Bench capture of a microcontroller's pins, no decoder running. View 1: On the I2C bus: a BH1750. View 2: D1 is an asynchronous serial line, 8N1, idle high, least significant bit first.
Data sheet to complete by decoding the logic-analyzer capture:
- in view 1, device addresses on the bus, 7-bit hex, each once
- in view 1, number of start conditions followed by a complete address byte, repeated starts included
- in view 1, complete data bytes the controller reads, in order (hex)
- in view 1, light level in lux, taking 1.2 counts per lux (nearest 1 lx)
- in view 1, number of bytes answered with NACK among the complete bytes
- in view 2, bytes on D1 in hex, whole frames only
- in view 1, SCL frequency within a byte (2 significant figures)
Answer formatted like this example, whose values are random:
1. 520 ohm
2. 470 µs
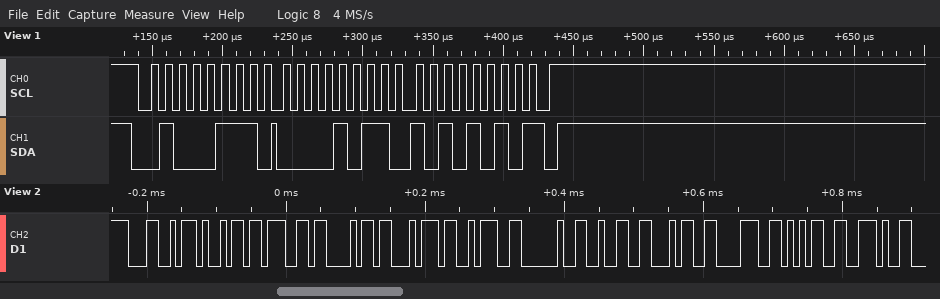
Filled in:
1. 0x23
2. 1
3. 0B AA
4. 2488 lx
5. 1
6. 0x4C 0x69 0x67 0x68 0x74 0x3A 0x20 0x32 0x34 0x38 0x35 0x2E
7. 100 kHz
